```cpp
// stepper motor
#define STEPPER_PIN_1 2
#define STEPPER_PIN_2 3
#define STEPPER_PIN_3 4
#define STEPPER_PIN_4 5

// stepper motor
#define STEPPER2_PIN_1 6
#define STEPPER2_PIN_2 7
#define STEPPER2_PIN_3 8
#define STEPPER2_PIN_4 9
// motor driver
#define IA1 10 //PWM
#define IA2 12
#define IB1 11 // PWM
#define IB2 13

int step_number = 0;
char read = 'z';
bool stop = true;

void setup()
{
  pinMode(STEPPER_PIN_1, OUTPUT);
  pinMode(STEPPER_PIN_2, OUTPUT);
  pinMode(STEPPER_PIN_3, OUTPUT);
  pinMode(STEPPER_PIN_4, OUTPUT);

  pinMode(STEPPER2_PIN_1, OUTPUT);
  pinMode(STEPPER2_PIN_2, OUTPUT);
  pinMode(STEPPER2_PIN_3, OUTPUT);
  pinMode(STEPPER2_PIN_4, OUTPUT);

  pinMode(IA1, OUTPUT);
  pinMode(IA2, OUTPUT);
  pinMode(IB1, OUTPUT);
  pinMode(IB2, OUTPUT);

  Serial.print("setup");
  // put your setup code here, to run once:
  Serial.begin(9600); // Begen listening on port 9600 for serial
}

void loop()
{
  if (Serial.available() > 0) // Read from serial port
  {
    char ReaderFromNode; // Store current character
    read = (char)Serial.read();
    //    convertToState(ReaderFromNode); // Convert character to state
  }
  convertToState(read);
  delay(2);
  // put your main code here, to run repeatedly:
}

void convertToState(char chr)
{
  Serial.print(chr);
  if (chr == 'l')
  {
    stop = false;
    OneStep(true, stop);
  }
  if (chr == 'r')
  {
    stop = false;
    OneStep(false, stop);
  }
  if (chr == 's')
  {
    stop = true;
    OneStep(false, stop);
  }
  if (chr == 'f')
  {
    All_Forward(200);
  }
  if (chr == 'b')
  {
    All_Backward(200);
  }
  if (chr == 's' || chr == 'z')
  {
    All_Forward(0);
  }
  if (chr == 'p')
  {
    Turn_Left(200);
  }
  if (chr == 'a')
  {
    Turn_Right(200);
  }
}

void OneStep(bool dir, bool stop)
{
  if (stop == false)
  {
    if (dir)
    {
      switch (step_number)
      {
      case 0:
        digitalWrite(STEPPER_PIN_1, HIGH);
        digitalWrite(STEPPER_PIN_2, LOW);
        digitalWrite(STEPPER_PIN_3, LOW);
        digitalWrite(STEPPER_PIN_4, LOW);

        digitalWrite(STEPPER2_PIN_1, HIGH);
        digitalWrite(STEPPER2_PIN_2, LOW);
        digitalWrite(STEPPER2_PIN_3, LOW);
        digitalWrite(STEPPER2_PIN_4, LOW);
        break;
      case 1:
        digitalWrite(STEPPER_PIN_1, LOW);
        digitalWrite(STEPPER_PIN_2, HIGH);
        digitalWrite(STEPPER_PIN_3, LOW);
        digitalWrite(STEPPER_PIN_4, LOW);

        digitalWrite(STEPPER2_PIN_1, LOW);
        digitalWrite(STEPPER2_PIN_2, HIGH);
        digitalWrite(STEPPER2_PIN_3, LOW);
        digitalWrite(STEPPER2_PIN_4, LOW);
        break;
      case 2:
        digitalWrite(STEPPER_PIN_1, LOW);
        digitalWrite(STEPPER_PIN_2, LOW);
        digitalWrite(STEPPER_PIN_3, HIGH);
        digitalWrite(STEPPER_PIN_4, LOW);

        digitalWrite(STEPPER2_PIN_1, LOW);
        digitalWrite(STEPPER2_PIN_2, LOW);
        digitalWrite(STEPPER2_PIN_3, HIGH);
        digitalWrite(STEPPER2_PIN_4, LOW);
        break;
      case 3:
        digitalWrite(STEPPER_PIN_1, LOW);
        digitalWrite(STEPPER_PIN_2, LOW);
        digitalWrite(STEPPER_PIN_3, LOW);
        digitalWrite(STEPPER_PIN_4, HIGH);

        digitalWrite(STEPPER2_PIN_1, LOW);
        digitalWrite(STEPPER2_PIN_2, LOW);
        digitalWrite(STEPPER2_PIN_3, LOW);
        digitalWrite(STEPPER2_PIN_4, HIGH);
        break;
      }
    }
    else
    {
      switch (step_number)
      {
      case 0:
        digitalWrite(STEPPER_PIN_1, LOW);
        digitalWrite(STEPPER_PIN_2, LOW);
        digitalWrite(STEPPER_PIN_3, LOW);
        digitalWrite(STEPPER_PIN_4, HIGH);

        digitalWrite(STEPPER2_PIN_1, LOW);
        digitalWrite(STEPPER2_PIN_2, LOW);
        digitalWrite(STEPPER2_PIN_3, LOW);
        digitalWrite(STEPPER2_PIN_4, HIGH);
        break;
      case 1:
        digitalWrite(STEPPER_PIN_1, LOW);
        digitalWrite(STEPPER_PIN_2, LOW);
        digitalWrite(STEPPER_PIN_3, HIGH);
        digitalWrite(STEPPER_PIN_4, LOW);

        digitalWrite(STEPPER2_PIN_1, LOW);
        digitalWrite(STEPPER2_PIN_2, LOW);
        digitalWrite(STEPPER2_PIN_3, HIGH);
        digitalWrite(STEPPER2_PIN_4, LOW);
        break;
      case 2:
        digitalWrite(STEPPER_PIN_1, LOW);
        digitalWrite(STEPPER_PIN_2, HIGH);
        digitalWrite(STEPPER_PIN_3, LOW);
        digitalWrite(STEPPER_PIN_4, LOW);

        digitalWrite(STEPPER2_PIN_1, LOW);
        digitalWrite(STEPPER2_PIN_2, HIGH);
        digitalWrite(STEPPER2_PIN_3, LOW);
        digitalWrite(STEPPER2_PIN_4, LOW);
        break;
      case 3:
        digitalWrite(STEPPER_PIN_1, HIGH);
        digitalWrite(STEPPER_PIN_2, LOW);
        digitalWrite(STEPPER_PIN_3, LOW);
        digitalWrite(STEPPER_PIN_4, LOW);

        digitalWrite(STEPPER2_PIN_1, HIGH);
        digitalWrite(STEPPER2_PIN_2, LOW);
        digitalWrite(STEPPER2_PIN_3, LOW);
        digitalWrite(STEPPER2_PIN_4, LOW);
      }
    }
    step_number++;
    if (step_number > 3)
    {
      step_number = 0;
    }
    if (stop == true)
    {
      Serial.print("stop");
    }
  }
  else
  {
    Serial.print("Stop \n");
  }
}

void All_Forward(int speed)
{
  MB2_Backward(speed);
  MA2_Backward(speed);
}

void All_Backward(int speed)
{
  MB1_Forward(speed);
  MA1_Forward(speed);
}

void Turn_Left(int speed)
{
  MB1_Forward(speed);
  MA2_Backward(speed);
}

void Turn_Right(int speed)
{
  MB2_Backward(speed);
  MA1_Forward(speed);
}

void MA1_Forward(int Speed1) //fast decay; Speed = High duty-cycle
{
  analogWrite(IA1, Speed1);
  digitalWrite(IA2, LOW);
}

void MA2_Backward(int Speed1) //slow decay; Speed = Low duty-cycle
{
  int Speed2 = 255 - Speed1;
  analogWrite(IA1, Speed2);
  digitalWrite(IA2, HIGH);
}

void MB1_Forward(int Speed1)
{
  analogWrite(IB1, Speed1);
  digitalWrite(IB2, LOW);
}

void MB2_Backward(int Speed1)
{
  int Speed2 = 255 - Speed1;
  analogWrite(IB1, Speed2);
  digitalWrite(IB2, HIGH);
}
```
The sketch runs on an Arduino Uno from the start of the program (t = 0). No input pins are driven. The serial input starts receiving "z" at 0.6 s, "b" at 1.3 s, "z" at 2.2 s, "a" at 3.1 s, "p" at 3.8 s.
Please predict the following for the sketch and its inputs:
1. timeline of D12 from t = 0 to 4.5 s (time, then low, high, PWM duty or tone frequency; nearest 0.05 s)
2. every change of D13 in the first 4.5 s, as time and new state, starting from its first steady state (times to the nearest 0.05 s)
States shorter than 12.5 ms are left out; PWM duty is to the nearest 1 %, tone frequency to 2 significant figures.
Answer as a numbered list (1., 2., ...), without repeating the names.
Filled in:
1. 0 s high; 1.3 s low; 2.2 s high; 3.1 s low; 3.8 s high
2. 0 s high; 1.3 s low; 2.2 s high; 3.8 s low
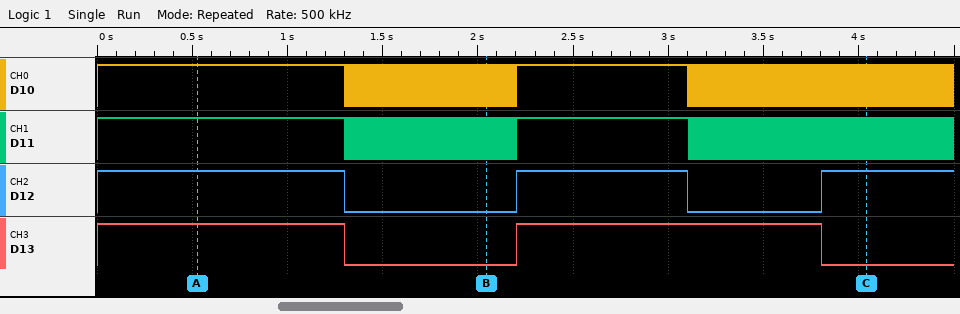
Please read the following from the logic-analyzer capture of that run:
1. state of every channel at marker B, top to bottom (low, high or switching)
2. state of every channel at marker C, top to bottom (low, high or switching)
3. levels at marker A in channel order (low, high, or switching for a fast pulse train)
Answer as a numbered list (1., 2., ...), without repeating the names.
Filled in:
1. D10 switching, D11 switching, D12 low, D13 low
2. D10 switching, D11 switching, D12 high, D13 low
3. D10 high, D11 high, D12 high, D13 high
